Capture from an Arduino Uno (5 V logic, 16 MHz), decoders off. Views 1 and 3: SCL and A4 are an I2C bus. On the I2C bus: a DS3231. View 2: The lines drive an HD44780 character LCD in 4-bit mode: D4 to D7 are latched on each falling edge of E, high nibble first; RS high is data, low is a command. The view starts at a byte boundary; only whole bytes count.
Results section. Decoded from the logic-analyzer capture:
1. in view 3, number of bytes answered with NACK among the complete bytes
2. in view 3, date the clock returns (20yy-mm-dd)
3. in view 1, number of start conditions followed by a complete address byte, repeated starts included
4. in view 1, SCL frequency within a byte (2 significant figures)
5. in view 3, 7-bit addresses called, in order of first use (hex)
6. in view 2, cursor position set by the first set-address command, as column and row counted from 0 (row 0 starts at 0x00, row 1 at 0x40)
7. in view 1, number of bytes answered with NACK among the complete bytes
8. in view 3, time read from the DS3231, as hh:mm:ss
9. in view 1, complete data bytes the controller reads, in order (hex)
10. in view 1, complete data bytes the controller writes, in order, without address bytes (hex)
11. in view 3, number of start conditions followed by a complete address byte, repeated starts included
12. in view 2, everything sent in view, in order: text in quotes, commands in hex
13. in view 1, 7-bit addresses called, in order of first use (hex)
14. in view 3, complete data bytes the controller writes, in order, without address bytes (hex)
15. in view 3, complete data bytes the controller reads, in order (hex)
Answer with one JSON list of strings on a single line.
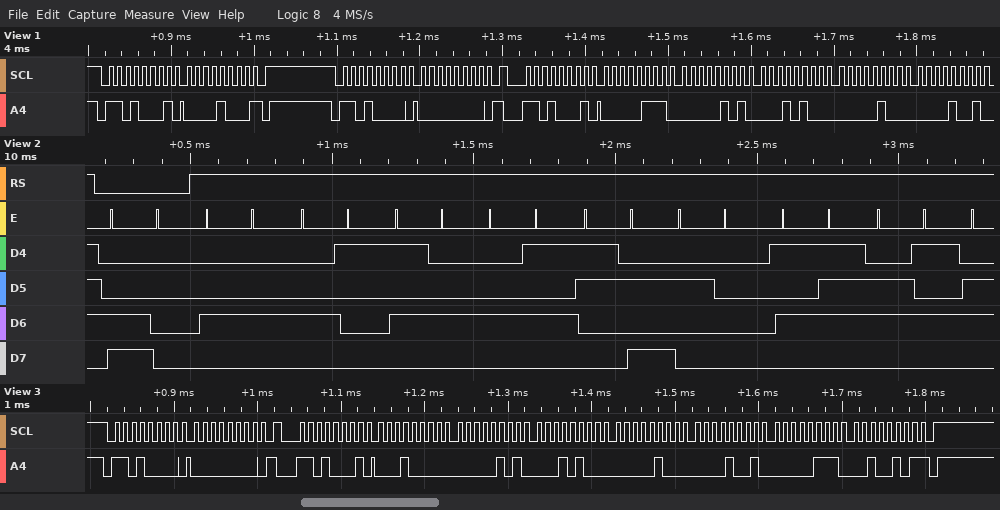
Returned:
["1", "2025-07-09", "3", "100 kHz", "0x68", "column 0, row 1", "1", "14:05:10", "08 07 05 14 04 09", "00", "2", "0xC0 \"DATE: We\"", "0x68", "00", "10 05 14 04 09 07 25"]
